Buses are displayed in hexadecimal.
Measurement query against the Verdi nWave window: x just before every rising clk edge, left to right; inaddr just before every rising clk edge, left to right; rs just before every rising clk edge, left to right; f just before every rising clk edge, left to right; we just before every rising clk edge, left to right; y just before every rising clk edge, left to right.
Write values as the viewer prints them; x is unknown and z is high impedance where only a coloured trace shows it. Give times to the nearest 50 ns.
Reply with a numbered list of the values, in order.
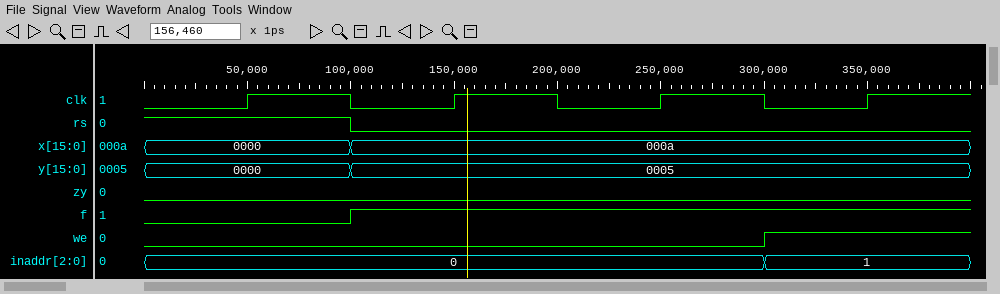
1. 0000, 000a, 000a, 000a
2. 0, 0, 0, 1
3. 1 0 0 0
4. 0 1 1 1
5. 0 0 0 1
6. 0000, 0005, 0005, 0005
